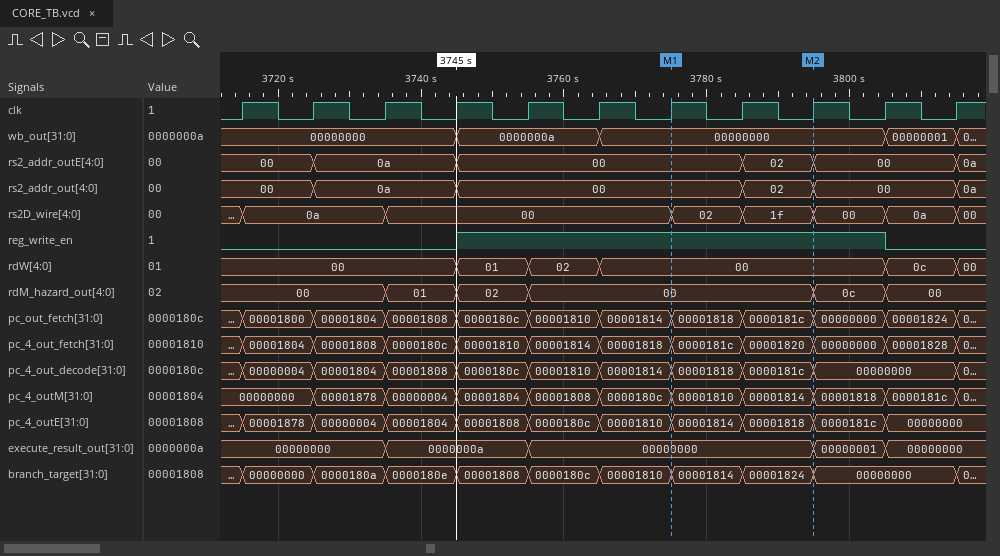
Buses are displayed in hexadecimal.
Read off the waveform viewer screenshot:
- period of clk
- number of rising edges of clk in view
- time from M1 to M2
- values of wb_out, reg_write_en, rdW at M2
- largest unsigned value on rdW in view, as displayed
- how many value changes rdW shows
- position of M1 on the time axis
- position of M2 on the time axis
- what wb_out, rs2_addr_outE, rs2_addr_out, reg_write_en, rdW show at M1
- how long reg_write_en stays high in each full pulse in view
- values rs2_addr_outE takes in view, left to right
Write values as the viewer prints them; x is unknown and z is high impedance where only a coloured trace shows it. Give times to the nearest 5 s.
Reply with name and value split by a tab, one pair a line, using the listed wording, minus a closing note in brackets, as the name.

period of clk	10 s
number of rising edges of clk in view	11
time from M1 to M2	20 s
values of wb_out, reg_write_en, rdW at M2	wb_out=00000000, reg_write_en=1, rdW=00
largest unsigned value on rdW in view, as displayed	0c
how many value changes rdW shows	5
position of M1 on the time axis	3775 s
position of M2 on the time axis	3795 s
what wb_out, rs2_addr_outE, rs2_addr_out, reg_write_en, rdW show at M1	wb_out=00000000, rs2_addr_outE=00, rs2_addr_out=00, reg_write_en=1, rdW=00
how long reg_write_en stays high in each full pulse in view	60 s
values rs2_addr_outE takes in view, left to right	00, 0a, 00, 02, 00, 0a
